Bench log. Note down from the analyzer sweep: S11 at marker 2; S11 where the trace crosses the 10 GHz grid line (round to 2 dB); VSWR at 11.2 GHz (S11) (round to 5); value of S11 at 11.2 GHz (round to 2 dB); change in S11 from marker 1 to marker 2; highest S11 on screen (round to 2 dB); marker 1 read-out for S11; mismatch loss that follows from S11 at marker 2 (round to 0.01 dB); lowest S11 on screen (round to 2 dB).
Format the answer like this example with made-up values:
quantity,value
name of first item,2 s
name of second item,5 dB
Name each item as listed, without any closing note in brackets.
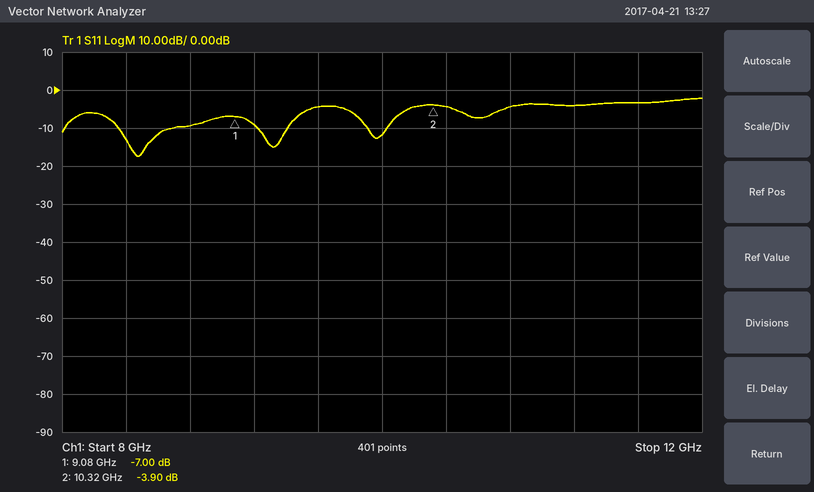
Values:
quantity,value
S11 at marker 2,-3.90 dB
S11 where the trace crosses the 10 GHz grid line,-12 dB
VSWR at 11.2 GHz (S11),5
value of S11 at 11.2 GHz,-4 dB
change in S11 from marker 1 to marker 2,3.10 dB
highest S11 on screen,-2 dB
marker 1 read-out for S11,-7.00 dB
mismatch loss that follows from S11 at marker 2,2.27 dB
lowest S11 on screen,-18 dB
